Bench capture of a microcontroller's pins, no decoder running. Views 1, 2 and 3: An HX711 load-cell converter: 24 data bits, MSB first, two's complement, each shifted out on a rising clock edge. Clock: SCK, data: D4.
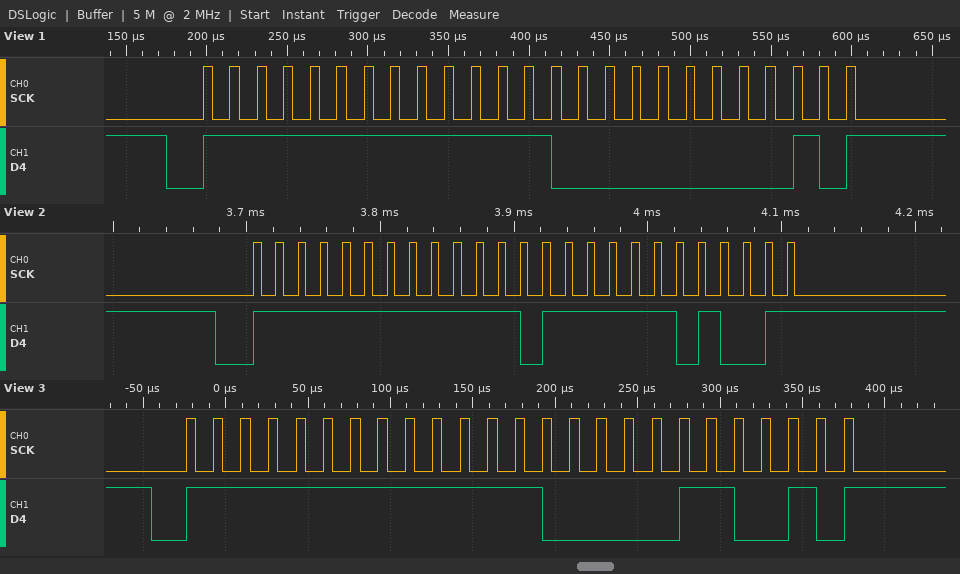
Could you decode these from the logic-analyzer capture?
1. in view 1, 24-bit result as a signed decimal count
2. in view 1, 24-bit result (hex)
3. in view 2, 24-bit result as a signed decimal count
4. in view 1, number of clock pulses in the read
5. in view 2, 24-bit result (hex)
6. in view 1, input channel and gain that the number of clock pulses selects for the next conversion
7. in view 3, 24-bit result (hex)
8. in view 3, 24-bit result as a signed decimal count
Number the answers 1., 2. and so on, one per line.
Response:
1. -2046
2. 0xFFF802
3. -2071
4. 25
5. 0xFFF7E9
6. channel A, gain 128
7. 0xFFF832
8. -1998
